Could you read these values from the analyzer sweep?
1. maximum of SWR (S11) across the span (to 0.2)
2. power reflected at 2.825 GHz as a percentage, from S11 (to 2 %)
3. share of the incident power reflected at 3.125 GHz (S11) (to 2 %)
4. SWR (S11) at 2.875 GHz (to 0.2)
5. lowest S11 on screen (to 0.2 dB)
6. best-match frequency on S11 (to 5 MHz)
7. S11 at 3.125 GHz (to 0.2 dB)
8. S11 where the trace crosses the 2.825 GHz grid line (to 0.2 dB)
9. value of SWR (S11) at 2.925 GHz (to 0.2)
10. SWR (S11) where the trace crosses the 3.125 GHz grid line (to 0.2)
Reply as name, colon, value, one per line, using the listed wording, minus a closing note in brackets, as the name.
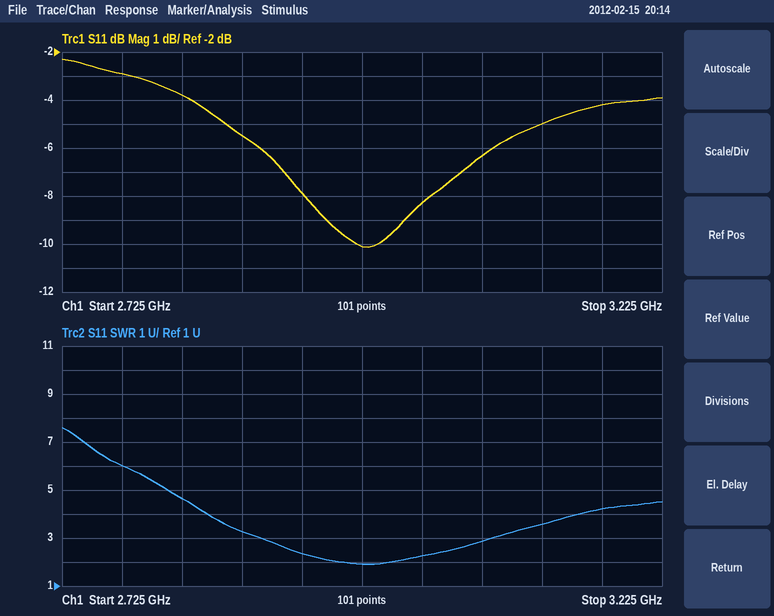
maximum of SWR (S11) across the span: 7.6
power reflected at 2.825 GHz as a percentage, from S11: 42 %
share of the incident power reflected at 3.125 GHz (S11): 32 %
SWR (S11) at 2.875 GHz: 3.2
lowest S11 on screen: -10.2 dB
best-match frequency on S11: 2.980 GHz
S11 at 3.125 GHz: -5.0 dB
S11 where the trace crosses the 2.825 GHz grid line: -3.8 dB
value of SWR (S11) at 2.925 GHz: 2.4
SWR (S11) where the trace crosses the 3.125 GHz grid line: 3.6
